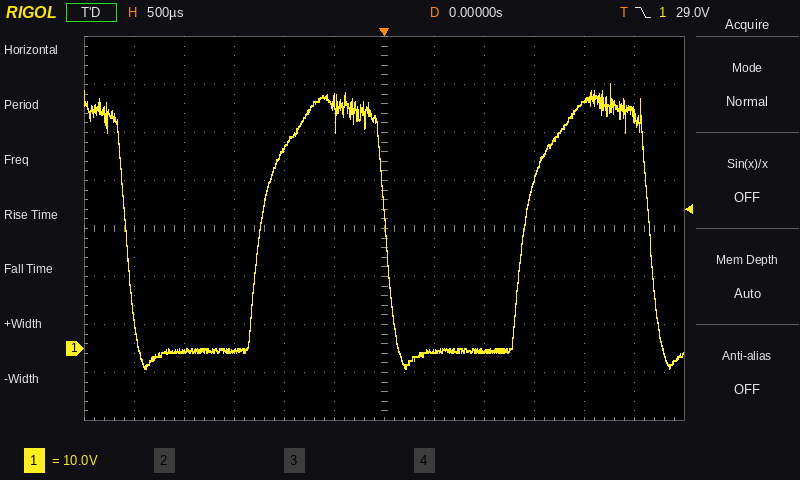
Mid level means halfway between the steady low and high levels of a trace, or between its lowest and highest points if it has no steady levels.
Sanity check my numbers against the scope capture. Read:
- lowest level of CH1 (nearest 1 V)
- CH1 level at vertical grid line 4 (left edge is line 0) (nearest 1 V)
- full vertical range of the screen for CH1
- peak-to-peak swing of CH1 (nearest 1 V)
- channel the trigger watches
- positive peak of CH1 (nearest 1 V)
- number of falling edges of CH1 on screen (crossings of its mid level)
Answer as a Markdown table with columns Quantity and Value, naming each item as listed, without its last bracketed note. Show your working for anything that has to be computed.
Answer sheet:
| Quantity | Value |
|---|---|
| lowest level of CH1 | -4 V |
| CH1 level at vertical grid line 4 (left edge is line 0) | 42 V |
| full vertical range of the screen for CH1 | 80 V |
| peak-to-peak swing of CH1 | 55 V − (-4 V) = 59 V |
| channel the trigger watches | CH1 |
| positive peak of CH1 | 55 V |
| number of falling edges of CH1 on screen | 3 |
